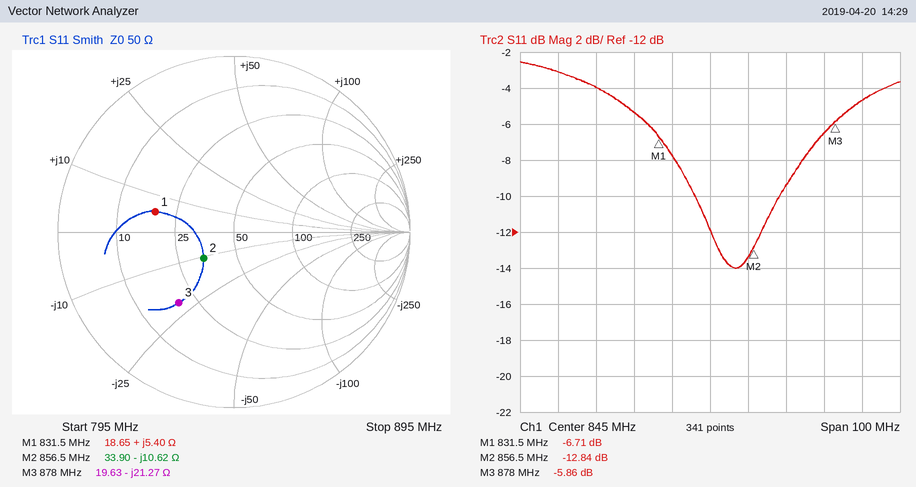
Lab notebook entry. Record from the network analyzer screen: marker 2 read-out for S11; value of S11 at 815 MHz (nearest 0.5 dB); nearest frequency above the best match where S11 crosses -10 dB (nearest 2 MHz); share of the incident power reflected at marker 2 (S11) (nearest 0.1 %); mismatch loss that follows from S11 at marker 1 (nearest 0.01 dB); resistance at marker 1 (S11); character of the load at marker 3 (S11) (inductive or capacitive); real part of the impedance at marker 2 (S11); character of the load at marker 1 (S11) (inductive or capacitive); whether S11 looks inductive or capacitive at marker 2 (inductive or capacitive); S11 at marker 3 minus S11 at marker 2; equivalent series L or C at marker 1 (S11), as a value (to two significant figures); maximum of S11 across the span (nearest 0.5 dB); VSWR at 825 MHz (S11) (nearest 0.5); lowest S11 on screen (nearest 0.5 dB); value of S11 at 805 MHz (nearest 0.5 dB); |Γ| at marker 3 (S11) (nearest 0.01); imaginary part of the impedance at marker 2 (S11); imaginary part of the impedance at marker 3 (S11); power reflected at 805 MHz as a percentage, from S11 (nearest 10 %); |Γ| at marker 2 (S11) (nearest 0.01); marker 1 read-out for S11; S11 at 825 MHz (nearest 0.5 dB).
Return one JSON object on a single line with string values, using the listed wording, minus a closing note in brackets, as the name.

{"marker 2 read-out for S11": "-12.84 dB", "value of S11 at 815 MHz": "-4.0 dB", "nearest frequency above the best match where S11 crosses -10 dB": "864 MHz", "share of the incident power reflected at marker 2 (S11)": "5.2 %", "mismatch loss that follows from S11 at marker 1": "1.04 dB", "resistance at marker 1": "18.65 Ω", "character of the load at marker 3 (S11)": "capacitive", "real part of the impedance at marker 2": "33.90 Ω", "character of the load at marker 1 (S11)": "inductive", "whether S11 looks inductive or capacitive at marker 2": "capacitive", "S11 at marker 3 minus S11 at marker 2": "6.98 dB", "equivalent series L or C at marker 1 (S11), as a value": "1.0 nH", "maximum of S11 across the span": "-2.5 dB", "VSWR at 825 MHz (S11)": "3.5", "lowest S11 on screen": "-14.0 dB", "value of S11 at 805 MHz": "-3.0 dB", "|Γ| at marker 3 (S11)": "0.51", "imaginary part of the impedance at marker 2": "-10.62 Ω", "imaginary part of the impedance at marker 3": "-21.27 Ω", "power reflected at 805 MHz as a percentage, from S11": "50 %", "|Γ| at marker 2 (S11)": "0.23", "marker 1 read-out for S11": "-6.71 dB", "S11 at 825 MHz": "-5.5 dB"}
